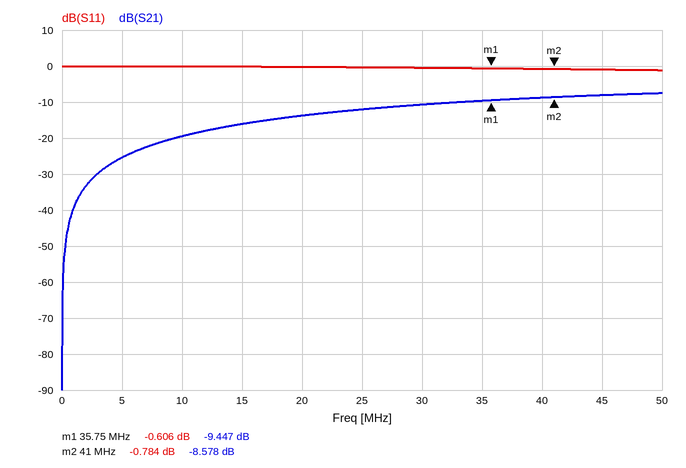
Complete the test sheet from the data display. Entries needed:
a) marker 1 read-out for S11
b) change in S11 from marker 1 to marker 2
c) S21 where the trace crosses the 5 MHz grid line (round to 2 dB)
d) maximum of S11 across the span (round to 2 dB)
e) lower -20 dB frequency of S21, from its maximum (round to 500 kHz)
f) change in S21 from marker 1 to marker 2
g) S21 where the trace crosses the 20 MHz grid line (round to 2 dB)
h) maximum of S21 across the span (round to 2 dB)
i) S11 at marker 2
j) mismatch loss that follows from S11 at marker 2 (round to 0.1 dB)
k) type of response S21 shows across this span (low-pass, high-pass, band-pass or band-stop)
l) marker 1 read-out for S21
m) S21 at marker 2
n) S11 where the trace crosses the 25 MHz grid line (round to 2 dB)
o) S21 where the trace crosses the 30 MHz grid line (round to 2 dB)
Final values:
-0.606 dB
-0.178 dB
-26 dB
0 dB
4.0 MHz
0.869 dB
-14 dB
-8 dB
-0.784 dB
7.8 dB
high-pass
-9.447 dB
-8.578 dB
0 dB
-10 dB
